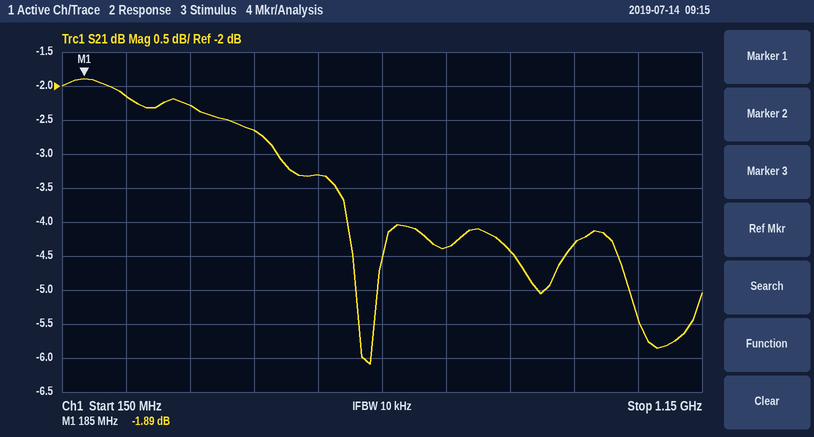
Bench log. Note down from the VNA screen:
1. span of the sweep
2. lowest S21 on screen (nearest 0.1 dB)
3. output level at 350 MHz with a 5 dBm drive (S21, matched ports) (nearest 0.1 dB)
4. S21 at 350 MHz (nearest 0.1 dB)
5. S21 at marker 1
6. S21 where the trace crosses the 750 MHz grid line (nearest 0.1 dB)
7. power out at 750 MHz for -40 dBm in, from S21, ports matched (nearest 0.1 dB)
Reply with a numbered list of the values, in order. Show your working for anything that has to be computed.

1. 1 GHz
2. -6.1 dB
3. 5 dBm + (-2.3 dB) = 2.7 dBm
4. -2.3 dB
5. -1.89 dB
6. -4.4 dB
7. -40 dBm + (-4.4 dB) = -44.4 dBm
